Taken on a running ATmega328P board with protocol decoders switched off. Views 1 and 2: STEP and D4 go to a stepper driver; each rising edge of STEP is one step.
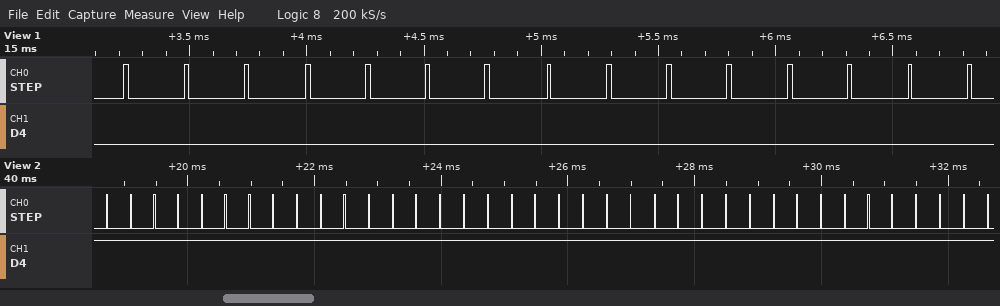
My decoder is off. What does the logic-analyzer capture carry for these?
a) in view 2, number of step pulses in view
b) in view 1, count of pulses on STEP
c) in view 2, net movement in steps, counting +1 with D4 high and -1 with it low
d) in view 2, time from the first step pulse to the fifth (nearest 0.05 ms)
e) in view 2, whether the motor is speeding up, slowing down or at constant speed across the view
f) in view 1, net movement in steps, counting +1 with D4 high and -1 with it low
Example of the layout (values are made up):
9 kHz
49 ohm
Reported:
38
15
+38
1.50 ms
constant speed
-15
